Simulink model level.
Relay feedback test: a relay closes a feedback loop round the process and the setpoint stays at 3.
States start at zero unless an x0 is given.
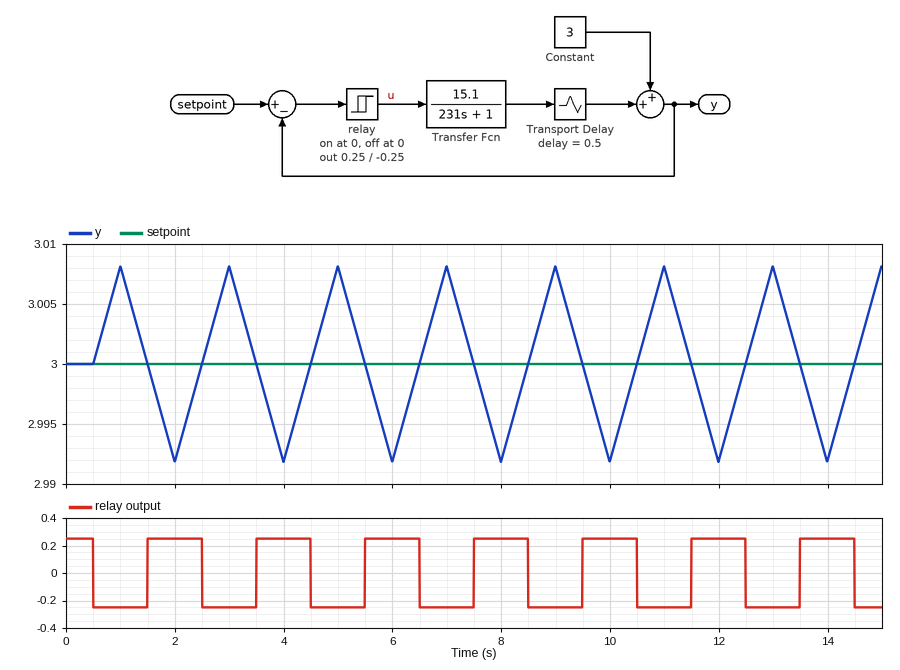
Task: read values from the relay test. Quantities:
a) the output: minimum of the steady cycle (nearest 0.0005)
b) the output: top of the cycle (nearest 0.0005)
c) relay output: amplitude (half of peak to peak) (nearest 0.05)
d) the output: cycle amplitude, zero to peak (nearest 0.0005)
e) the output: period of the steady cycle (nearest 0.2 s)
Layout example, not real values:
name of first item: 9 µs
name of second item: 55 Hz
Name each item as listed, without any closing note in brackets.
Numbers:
the output: minimum of the steady cycle: 2.9920
the output: top of the cycle: 3.0080
relay output: amplitude (half of peak to peak): 0.25
the output: cycle amplitude, zero to peak: 0.0080
the output: period of the steady cycle: 2.0 s
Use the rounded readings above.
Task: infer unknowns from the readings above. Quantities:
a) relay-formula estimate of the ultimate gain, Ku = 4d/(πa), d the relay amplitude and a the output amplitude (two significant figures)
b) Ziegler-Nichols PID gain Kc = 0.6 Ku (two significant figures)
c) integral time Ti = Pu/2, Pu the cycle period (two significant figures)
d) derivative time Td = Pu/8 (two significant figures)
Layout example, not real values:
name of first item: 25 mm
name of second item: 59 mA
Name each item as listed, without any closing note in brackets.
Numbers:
relay-formula estimate of the ultimate gain, Ku = 4d/(πa), d the relay amplitude and a the output amplitude: 40
Ziegler-Nichols PID gain Kc = 0.6 Ku: 24
integral time Ti = Pu/2, Pu the cycle period: 1.0 s
derivative time Td = Pu/8: 0.25 s
